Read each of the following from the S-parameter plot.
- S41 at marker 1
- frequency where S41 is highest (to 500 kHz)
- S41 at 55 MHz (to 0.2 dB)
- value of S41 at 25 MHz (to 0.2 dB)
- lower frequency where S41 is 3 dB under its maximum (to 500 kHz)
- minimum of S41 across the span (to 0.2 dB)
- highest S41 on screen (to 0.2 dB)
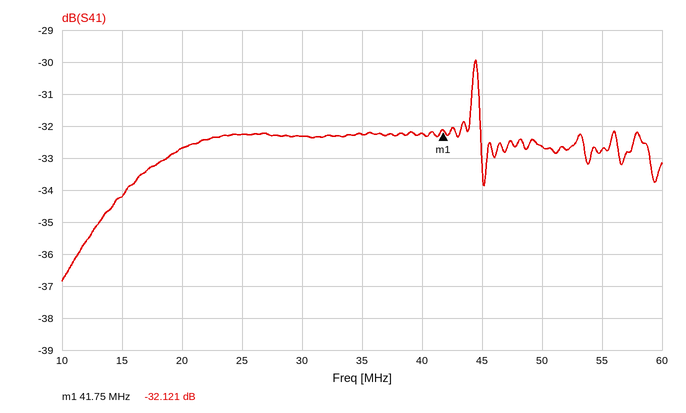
-32.121 dB
44.5 MHz
-32.8 dB
-32.2 dB
19.0 MHz
-36.8 dB
-30.0 dB
